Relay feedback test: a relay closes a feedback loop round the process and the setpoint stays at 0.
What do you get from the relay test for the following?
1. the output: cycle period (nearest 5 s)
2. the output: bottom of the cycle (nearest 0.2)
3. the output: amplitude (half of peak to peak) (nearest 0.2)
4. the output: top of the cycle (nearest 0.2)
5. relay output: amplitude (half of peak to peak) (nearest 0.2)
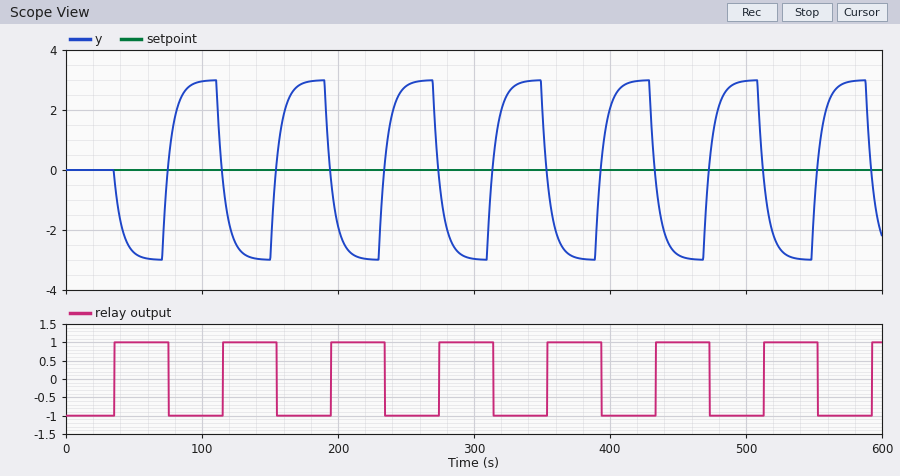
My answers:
80 s
-3.0
3.0
3.0
1.0
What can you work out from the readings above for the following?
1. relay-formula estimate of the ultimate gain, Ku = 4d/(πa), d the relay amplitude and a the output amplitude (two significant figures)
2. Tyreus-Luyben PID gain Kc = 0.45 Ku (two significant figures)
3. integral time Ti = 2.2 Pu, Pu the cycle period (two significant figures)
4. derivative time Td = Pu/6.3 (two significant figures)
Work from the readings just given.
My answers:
0.42
0.19
180 s
13 s
